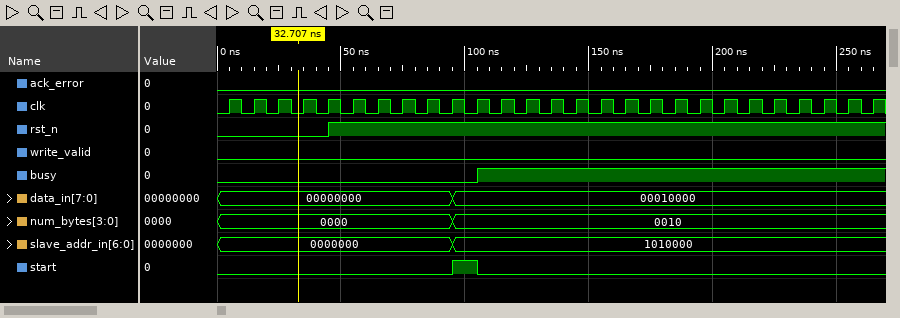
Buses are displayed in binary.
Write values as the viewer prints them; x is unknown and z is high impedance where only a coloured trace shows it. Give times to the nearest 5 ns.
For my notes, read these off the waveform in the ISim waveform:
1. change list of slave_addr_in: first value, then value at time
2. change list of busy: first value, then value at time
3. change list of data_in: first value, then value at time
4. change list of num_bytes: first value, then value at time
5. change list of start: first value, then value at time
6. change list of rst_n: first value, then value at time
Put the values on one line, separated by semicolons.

0000000, 1010000 at 95 ns; 0, 1 at 105 ns; 00000000, 00010000 at 95 ns; 0000, 0010 at 95 ns; 0, 1 at 95 ns, 0 at 105 ns; 0, 1 at 45 ns
